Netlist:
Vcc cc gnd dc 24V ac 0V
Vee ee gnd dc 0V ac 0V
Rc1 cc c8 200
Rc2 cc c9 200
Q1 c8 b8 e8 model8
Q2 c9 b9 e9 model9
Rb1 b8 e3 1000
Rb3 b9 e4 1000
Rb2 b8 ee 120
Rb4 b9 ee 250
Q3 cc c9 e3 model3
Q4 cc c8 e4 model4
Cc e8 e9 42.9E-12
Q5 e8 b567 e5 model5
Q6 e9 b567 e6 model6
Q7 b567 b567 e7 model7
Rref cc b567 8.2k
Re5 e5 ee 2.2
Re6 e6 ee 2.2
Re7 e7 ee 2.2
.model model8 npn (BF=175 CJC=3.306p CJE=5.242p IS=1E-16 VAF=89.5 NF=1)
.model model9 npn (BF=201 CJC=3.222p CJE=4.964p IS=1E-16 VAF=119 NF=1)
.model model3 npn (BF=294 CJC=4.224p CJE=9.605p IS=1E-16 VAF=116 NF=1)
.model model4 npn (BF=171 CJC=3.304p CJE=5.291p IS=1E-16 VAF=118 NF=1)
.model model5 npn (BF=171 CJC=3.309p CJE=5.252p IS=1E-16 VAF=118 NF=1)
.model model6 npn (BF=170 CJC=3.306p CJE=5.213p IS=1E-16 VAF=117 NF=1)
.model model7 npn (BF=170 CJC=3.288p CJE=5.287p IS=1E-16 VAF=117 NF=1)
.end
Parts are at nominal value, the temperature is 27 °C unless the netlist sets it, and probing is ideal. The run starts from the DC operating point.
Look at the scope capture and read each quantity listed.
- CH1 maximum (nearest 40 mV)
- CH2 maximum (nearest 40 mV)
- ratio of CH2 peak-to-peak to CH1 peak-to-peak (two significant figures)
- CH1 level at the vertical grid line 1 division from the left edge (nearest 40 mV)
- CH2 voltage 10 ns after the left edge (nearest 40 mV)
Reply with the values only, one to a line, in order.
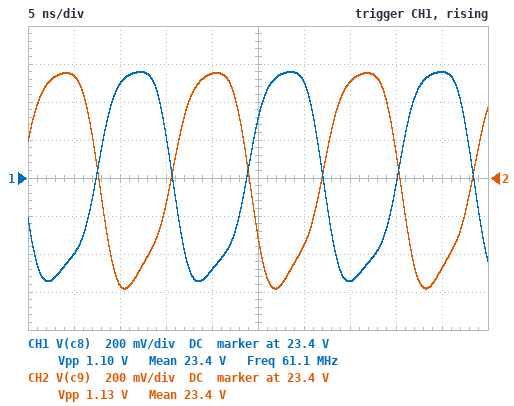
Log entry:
23.96 V
23.96 V
1.0
23.00 V
22.84 V
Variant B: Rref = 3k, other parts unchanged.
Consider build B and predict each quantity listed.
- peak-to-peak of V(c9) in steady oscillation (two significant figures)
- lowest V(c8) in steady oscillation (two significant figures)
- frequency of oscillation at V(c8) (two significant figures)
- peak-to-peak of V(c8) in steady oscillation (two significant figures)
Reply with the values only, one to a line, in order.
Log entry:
3.5 V
21 V
63 MHz
3.3 V
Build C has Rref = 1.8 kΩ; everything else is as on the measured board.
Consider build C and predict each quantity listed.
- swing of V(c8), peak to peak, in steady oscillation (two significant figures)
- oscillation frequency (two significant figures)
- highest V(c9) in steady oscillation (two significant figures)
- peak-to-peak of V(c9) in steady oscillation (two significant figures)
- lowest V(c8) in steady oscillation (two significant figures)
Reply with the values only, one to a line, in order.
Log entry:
5.7 V
63 MHz
24 V
5.9 V
18 V
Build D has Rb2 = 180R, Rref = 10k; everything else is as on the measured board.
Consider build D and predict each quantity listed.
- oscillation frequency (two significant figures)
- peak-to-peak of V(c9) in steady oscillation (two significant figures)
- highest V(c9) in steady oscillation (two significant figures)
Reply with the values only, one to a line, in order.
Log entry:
55 MHz
930 mV
24 V
